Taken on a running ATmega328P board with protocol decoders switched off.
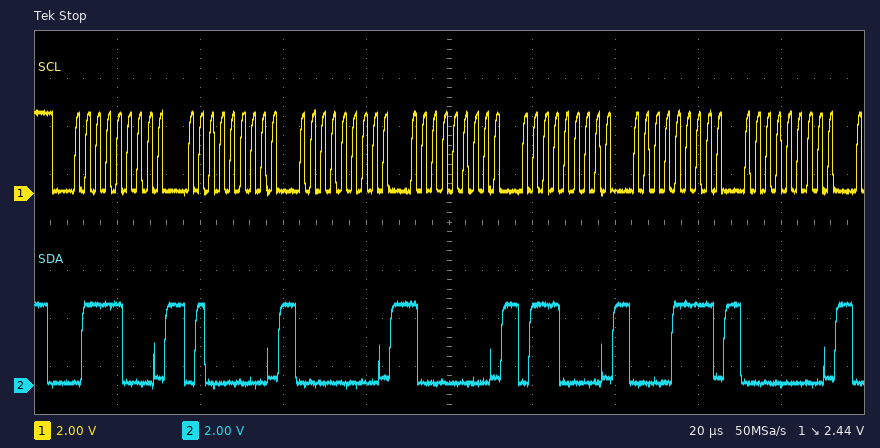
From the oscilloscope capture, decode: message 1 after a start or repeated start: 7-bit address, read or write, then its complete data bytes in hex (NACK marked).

0x3C write: 40 00 80 70 0F 00
